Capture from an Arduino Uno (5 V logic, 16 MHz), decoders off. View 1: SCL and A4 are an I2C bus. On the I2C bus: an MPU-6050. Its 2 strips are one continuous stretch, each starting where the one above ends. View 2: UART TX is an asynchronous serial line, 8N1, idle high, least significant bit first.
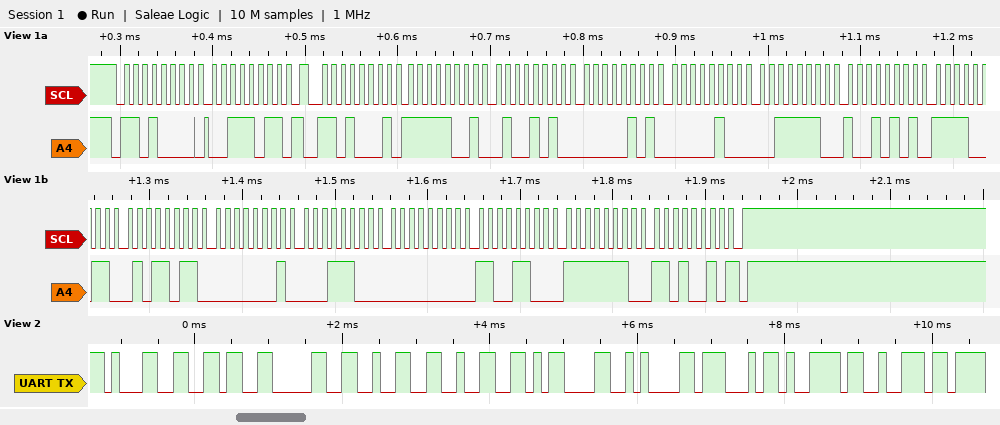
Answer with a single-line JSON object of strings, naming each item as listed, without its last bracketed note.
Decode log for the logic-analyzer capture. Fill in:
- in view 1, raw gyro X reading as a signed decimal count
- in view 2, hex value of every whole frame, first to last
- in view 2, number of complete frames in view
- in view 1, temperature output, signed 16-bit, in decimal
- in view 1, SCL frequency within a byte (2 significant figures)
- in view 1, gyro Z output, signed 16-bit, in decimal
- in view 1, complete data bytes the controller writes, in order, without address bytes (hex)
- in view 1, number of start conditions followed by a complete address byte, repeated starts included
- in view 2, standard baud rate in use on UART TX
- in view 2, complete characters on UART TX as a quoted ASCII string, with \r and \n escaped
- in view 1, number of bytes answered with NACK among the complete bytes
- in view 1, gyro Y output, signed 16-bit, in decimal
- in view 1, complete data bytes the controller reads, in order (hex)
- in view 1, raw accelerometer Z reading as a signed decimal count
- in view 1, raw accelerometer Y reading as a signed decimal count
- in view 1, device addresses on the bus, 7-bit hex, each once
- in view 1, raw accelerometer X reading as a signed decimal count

{"in view 1, raw gyro X reading as a signed decimal count": "284", "in view 2, hex value of every whole frame, first to last": "31 36 30 32 32 0D 0A 47 79 72", "in view 2, number of complete frames in view": "10", "in view 1, temperature output, signed 16-bit, in decimal": "-3237", "in view 1, SCL frequency within a byte": "100 kHz", "in view 1, gyro Z output, signed 16-bit, in decimal": "-302", "in view 1, complete data bytes the controller writes, in order, without address bytes": "3B", "in view 1, number of start conditions followed by a complete address byte, repeated starts included": "2", "in view 2, standard baud rate in use on UART TX": "9600 baud", "in view 2, complete characters on UART TX as a quoted ASCII string, with \\r and \\n escaped": "\"16022\\r\\nGyr\"", "in view 1, number of bytes answered with NACK among the complete bytes": "1", "in view 1, gyro Y output, signed 16-bit, in decimal": "204", "in view 1, complete data bytes the controller reads, in order": "F9 4A 05 04 3E 95 F3 5B 01 1C 00 CC FE D2", "in view 1, raw accelerometer Z reading as a signed decimal count": "16021", "in view 1, raw accelerometer Y reading as a signed decimal count": "1284", "in view 1, device addresses on the bus, 7-bit hex, each once": "0x68", "in view 1, raw accelerometer X reading as a signed decimal count": "-1718"}
